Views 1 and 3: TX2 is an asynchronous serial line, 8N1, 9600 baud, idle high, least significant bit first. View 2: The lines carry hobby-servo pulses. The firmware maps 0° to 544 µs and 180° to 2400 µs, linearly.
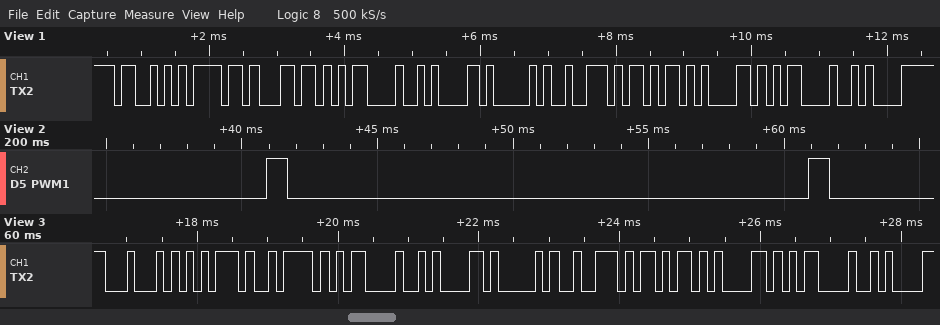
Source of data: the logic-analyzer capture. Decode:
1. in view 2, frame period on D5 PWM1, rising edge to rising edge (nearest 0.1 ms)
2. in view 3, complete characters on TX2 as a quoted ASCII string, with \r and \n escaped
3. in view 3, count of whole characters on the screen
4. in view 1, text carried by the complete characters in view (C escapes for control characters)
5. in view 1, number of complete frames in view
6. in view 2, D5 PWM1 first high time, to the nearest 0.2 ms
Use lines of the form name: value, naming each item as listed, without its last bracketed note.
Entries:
in view 2, frame period on D5 PWM1, rising edge to rising edge: 20.0 ms
in view 3, complete characters on TX2 as a quoted ASCII string, with \r and \n escaped: "Duz\r\nArka\r\n"
in view 3, count of whole characters on the screen: 11
in view 1, text carried by the complete characters in view: "Sol\r\nArka\r\n"
in view 1, number of complete frames in view: 11
in view 2, D5 PWM1 first high time, to the nearest 0.2 ms: 0.8 ms
